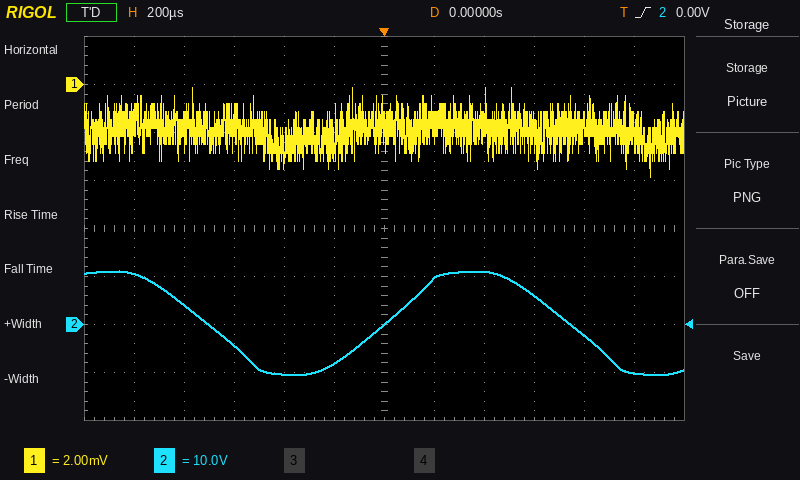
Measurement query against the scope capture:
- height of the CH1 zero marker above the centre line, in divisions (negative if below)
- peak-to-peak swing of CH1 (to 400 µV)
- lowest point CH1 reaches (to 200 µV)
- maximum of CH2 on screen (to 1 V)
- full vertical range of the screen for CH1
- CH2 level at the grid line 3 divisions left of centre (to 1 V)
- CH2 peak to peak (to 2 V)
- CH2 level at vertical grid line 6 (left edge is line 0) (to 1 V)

+3.0 div
3.6 mV
-3.8 mV
11 V
16 mV
-4 V
22 V
0 V
